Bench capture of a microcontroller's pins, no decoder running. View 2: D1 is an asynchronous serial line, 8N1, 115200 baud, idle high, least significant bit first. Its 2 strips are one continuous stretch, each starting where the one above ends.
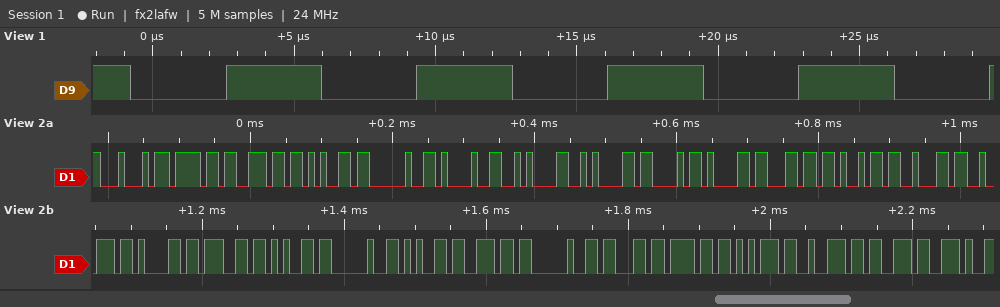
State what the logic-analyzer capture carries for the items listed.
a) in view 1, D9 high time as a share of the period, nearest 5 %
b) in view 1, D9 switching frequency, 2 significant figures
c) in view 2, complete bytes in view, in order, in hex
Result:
50 %
150 kHz
44 6F 6E 65 20 21 0A 0A 43 61 6C 69 62 72 61 67 65 20 65 6E 20 63 6F 75 72 73 2E
